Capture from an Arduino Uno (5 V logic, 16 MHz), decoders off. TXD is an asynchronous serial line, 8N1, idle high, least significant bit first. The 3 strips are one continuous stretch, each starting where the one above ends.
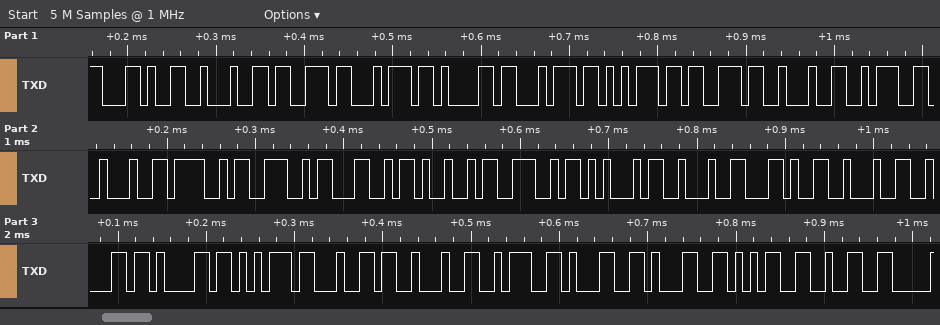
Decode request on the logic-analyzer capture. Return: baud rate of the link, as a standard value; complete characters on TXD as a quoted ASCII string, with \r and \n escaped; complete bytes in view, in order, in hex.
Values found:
115200 baud
",\"status\":\"ONLINE\",\"baud\":1152"
2C 22 73 74 61 74 75 73 22 3A 22 4F 4E 4C 49 4E 45 22 2C 22 62 61 75 64 22 3A 31 31 35 32
